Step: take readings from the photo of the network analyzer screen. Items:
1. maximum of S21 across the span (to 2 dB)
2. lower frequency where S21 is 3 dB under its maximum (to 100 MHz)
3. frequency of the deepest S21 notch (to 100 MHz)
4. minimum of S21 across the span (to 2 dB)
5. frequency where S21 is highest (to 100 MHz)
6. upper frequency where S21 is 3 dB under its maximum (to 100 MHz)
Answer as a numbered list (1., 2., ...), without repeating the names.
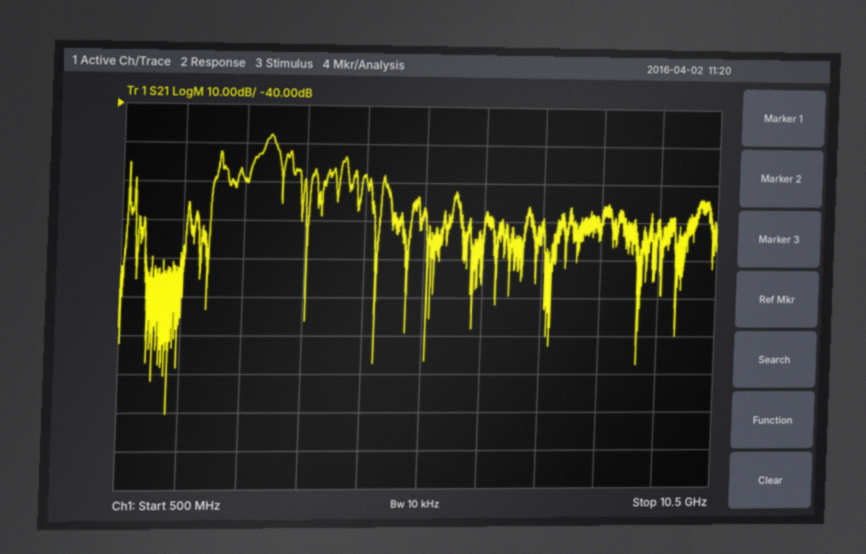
1. -48 dB
2. 2.8 GHz
3. 1.3 GHz
4. -120 dB
5. 2.9 GHz
6. 3.0 GHz
